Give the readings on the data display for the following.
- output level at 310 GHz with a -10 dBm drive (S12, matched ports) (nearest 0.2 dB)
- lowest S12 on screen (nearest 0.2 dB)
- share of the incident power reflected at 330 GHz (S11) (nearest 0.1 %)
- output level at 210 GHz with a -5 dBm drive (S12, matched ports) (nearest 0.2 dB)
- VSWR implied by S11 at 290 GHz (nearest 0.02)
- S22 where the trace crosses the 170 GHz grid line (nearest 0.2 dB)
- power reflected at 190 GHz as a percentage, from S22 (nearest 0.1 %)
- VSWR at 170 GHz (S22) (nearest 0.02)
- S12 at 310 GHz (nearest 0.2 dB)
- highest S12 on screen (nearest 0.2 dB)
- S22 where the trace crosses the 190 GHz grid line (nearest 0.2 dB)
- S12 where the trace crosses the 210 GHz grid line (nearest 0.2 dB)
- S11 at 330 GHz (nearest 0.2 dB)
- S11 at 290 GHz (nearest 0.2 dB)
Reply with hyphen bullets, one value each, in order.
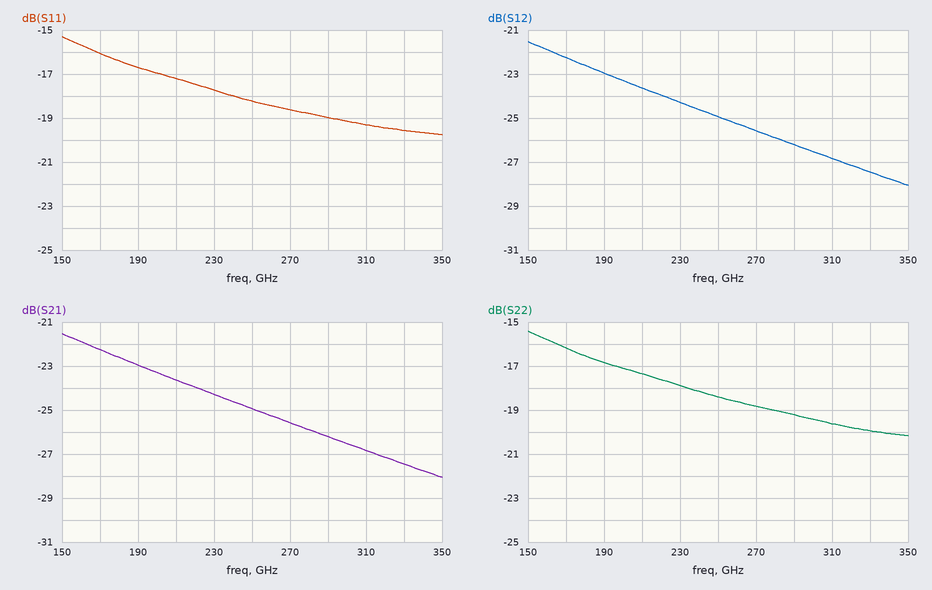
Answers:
- -36.8 dBm
- -28.0 dB
- 1.1 %
- -28.6 dBm
- 1.26
- -16.2 dB
- 2.1 %
- 1.36
- -26.8 dB
- -21.6 dB
- -16.8 dB
- -23.6 dB
- -19.6 dB
- -19.0 dB
